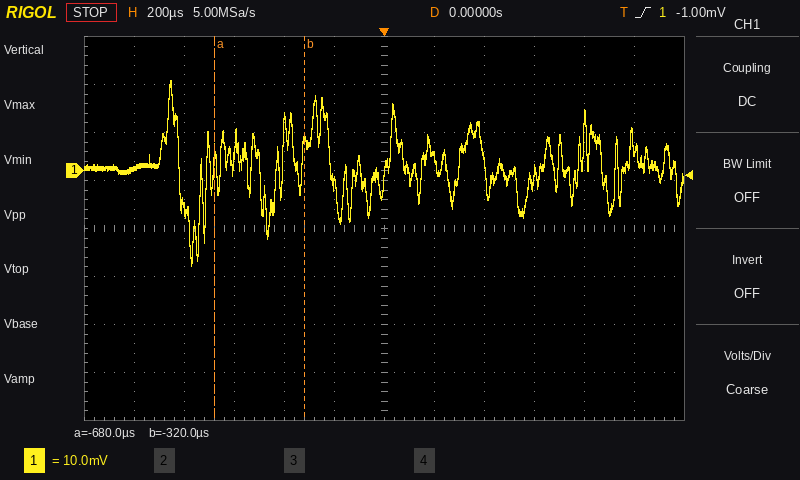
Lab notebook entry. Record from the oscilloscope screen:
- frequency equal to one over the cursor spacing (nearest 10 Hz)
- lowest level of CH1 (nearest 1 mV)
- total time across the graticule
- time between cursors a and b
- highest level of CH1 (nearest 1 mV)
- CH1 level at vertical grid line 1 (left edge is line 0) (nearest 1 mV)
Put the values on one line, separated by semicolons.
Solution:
2.78 kHz; -20 mV; 2.4 ms; 360 µs; 19 mV; 1 mV
